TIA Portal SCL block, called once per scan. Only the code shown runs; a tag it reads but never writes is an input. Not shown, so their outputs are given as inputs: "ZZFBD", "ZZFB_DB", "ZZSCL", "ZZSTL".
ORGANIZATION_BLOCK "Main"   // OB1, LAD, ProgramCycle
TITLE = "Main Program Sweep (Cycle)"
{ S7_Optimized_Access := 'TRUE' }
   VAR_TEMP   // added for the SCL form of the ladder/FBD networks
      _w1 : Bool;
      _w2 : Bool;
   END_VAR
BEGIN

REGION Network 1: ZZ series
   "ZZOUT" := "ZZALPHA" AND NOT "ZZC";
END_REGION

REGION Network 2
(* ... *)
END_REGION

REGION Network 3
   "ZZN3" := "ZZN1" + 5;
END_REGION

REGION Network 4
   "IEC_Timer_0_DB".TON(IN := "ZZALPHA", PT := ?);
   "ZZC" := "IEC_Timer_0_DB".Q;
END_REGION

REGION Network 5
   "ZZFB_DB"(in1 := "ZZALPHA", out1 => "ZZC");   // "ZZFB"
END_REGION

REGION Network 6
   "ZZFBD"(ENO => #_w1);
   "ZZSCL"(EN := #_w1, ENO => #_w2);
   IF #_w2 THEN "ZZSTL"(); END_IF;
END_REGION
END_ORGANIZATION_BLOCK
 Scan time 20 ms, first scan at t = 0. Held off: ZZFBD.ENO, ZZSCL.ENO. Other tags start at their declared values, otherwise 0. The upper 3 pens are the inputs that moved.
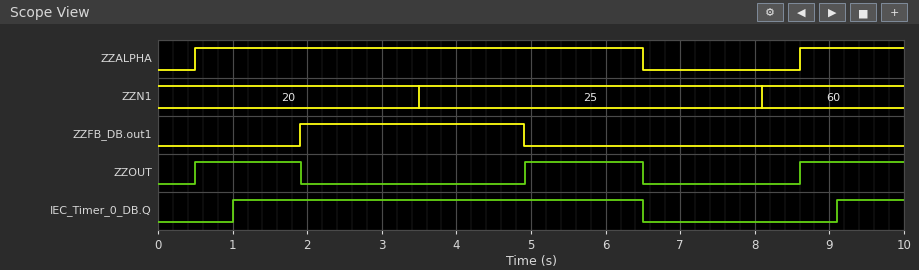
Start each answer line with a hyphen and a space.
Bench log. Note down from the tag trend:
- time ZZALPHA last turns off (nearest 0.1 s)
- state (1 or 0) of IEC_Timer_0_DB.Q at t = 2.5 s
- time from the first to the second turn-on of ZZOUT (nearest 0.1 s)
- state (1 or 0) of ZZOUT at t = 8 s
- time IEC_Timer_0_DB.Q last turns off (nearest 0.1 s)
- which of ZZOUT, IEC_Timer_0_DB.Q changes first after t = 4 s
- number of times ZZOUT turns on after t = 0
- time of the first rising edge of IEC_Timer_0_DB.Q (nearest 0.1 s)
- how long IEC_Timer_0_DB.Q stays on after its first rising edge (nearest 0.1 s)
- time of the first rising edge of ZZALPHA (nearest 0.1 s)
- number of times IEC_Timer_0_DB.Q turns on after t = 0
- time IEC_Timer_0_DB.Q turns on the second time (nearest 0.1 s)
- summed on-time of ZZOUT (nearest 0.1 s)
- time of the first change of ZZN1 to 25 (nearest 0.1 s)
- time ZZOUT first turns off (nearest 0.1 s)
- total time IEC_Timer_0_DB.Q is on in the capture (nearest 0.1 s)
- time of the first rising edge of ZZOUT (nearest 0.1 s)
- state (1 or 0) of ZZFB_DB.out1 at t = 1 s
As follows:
- 6.5 s
- 1
- 4.4 s
- 0
- 6.5 s
- ZZOUT
- 3
- 1.0 s
- 5.5 s
- 0.5 s
- 2
- 9.1 s
- 4.4 s
- 3.5 s
- 1.9 s
- 6.4 s
- 0.5 s
- 0
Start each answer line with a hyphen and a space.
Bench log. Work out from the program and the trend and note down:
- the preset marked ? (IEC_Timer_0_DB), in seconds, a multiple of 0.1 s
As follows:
- 0.5 s
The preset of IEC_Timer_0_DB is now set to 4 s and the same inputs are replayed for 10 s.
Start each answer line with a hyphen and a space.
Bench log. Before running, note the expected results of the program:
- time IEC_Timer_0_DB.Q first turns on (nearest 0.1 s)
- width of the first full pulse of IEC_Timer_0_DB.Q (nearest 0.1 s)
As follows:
- 4.5 s
- 2.0 s
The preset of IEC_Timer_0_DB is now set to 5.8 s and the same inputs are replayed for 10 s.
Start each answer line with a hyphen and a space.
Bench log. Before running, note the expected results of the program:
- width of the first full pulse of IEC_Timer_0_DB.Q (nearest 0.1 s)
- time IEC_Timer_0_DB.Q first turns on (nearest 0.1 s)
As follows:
- 0.2 s
- 6.3 s
